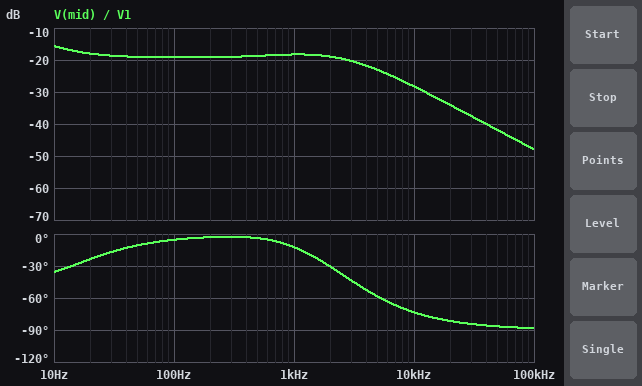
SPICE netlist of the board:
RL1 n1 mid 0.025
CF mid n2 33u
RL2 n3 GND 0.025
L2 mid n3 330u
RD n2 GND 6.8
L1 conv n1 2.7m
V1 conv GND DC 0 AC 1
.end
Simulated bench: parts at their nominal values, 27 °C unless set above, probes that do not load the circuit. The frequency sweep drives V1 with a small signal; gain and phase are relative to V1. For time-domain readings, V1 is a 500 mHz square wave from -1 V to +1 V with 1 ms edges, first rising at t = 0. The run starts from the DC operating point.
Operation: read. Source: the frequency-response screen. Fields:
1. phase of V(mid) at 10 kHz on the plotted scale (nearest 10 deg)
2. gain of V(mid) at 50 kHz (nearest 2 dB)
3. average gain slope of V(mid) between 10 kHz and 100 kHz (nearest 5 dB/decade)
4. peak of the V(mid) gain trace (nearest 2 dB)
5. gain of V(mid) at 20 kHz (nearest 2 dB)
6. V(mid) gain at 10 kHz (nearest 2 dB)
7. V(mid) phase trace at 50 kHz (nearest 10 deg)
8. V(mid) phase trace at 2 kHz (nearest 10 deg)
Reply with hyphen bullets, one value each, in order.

- -70 deg
- -42 dB
- -20 dB/decade
- -16 dB
- -34 dB
- -28 dB
- -90 deg
- -30 deg
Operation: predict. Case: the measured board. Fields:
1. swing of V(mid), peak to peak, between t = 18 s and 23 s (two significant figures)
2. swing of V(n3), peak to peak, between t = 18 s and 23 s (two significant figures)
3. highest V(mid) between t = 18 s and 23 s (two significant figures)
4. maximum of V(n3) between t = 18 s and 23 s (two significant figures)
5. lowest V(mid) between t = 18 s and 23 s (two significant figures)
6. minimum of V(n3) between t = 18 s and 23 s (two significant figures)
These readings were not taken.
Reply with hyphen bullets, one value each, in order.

- 1.0 V
- 1.0 V
- 500 mV
- 500 mV
- -500 mV
- -500 mV
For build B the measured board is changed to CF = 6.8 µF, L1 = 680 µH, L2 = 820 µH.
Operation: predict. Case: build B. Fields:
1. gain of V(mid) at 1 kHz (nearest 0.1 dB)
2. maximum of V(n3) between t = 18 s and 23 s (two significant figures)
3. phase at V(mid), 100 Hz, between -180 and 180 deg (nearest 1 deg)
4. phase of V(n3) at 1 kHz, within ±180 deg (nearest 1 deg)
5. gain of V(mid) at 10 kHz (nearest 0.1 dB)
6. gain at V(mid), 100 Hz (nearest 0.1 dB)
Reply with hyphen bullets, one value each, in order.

- -4.4 dB
- 500 mV
- 0 deg
- -91 deg
- -15.0 dB
- -5.2 dB
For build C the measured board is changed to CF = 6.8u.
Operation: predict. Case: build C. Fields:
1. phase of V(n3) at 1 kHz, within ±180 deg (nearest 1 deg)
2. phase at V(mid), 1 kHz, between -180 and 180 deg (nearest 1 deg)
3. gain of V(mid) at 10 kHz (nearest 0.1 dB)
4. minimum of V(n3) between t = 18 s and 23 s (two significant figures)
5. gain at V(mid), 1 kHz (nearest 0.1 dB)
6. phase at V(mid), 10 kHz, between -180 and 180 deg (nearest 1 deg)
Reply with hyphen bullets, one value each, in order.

- -91 deg
- -2 deg
- -27.0 dB
- -500 mV
- -18.6 dB
- -86 deg
